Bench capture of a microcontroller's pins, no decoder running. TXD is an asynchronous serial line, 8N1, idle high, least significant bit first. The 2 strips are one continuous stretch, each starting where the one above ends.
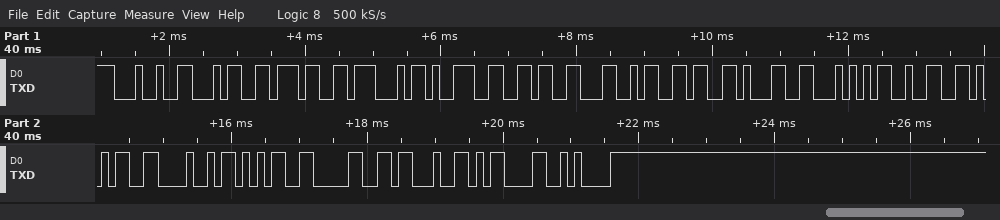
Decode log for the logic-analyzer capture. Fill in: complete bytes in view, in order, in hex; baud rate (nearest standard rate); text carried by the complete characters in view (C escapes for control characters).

0x24 0x34 0x37 0x47 0x39 0x36 0x4C 0x36 0x31 0x54 0x32 0x35 0x48 0x35 0x30 0x23 0x0D 0x0A
9600 baud
"$47G96L61T25H50#\r\n"
